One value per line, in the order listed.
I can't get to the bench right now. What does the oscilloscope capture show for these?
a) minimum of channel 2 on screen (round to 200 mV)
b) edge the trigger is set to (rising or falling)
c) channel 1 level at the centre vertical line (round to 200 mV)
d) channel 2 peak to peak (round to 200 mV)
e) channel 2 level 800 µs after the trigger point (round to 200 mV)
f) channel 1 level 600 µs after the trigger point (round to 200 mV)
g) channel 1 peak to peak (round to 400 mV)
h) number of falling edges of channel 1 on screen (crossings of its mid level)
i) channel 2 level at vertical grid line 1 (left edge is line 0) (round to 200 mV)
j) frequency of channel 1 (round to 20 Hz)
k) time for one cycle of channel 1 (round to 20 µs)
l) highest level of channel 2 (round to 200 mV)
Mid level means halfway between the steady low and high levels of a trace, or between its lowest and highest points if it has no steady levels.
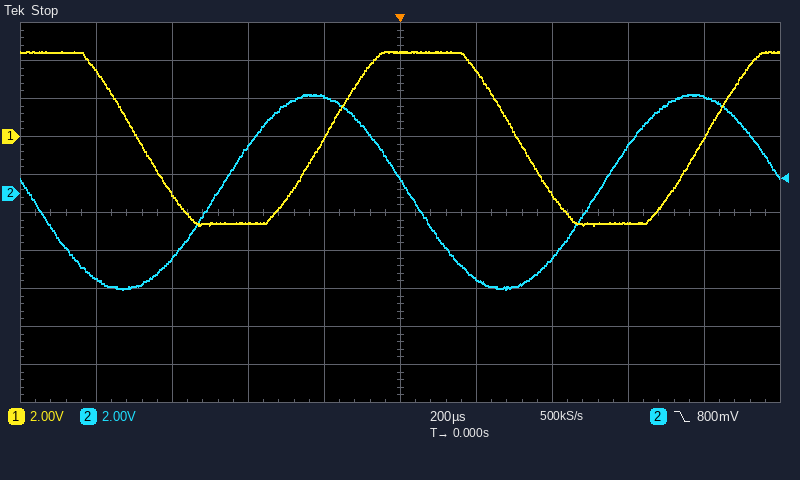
-5.0 V
falling
4.4 V
10.2 V
5.0 V
-4.6 V
9.2 V
2
-4.4 V
1.00 kHz
1.00 ms
5.2 V
